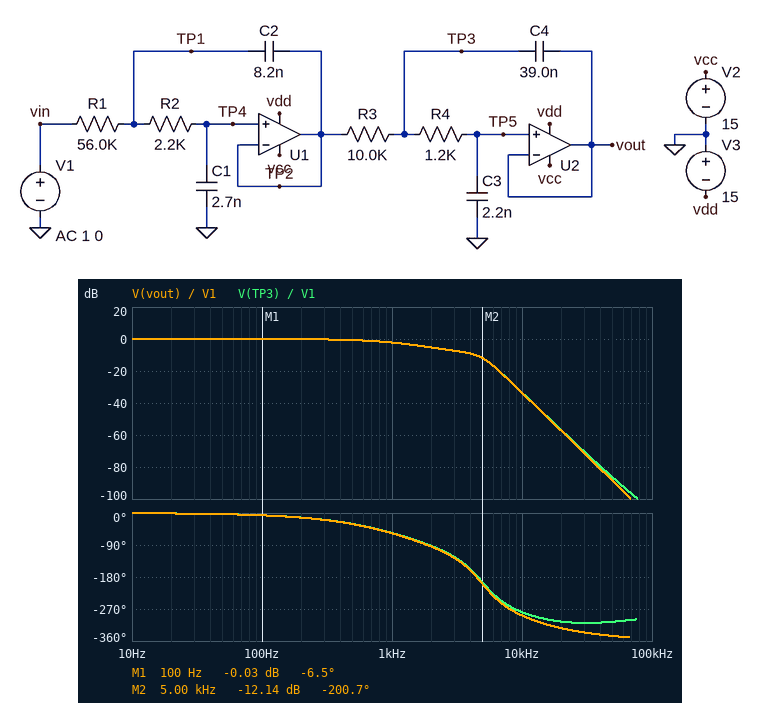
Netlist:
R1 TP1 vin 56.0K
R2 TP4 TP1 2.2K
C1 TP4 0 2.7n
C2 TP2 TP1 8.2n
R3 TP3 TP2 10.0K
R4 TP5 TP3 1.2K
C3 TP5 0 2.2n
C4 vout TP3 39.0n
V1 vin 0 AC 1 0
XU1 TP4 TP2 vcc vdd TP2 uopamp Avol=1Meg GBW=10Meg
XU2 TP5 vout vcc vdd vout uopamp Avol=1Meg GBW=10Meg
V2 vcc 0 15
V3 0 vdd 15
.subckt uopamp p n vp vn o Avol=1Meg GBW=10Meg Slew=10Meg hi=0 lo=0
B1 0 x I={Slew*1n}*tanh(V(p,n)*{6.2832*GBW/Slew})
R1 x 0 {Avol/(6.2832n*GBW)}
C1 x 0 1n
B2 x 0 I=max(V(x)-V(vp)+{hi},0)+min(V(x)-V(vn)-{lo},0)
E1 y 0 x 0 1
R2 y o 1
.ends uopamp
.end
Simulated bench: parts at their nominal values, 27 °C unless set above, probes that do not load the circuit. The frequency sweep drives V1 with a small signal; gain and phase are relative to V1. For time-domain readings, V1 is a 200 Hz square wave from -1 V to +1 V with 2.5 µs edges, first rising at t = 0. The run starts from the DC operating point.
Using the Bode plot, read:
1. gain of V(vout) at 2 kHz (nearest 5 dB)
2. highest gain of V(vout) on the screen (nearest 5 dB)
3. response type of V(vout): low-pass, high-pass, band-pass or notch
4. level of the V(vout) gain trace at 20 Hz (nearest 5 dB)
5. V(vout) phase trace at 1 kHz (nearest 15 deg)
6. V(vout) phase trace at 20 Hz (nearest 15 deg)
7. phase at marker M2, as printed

-5 dB
0 dB
low-pass
0 dB
-60 deg
0 deg
-200.7 deg
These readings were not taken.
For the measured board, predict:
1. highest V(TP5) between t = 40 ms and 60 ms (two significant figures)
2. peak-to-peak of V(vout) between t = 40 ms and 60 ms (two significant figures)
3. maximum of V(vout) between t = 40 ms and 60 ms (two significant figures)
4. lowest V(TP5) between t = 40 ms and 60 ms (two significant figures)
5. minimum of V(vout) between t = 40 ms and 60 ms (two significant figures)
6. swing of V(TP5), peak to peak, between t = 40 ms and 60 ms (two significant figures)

1.0 V
2.0 V
1.0 V
-1.0 V
-1.0 V
2.0 V
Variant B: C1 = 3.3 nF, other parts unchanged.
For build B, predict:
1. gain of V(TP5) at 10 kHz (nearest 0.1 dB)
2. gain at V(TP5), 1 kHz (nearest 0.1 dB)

-35.5 dB
-3.2 dB
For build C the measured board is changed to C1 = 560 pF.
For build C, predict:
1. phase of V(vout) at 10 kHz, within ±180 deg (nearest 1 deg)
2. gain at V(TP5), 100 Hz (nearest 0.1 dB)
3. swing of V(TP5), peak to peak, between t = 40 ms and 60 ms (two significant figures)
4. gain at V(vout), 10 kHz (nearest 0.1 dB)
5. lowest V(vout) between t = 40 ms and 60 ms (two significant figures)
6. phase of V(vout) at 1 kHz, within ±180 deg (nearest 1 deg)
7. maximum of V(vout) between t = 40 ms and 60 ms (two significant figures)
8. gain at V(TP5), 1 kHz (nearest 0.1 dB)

85 deg
0 dB
3.1 V
-18.4 dB
-1.6 V
-21 deg
1.6 V
0.3 dB
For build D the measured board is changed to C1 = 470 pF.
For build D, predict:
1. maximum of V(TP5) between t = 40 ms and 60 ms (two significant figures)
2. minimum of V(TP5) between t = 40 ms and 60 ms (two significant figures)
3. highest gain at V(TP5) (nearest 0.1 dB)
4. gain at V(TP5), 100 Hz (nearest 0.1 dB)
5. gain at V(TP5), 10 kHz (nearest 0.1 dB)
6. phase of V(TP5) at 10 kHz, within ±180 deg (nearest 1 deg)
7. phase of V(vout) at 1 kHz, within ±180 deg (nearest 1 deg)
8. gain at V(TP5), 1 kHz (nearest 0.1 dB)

1.6 V
-1.6 V
3.2 dB
0 dB
-16.5 dB
89 deg
-19 deg
0.3 dB
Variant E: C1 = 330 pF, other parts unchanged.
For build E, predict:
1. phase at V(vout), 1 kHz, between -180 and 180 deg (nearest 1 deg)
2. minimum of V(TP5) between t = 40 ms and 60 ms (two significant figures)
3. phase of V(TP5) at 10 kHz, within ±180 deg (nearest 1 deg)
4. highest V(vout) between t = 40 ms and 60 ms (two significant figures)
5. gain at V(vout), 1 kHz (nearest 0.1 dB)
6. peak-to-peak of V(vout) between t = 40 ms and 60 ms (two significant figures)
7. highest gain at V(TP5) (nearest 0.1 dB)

-16 deg
-1.7 V
101 deg
1.7 V
0.3 dB
3.4 V
3.8 dB
